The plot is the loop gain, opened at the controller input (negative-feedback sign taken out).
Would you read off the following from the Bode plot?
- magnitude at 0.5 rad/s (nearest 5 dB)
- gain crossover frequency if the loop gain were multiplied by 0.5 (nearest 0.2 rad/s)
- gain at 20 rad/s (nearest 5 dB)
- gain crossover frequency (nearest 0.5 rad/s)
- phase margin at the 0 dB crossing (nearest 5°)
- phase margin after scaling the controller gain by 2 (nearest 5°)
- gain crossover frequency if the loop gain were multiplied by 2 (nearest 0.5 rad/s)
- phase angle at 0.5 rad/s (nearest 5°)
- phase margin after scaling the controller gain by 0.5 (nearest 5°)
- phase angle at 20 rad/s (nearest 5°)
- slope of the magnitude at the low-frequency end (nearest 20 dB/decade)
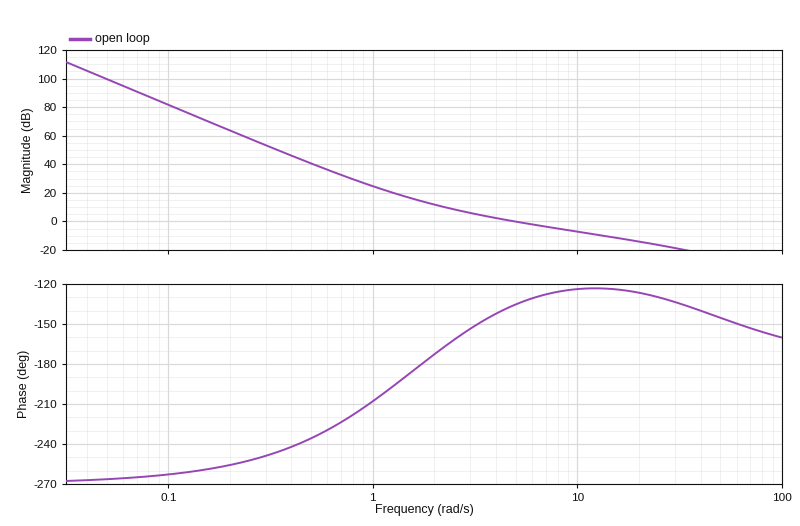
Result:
40 dB
3.0 rad/s
-15 dB
5.0 rad/s
45°
55°
9.0 rad/s
-235°
25°
-125°
-60 dB/decade
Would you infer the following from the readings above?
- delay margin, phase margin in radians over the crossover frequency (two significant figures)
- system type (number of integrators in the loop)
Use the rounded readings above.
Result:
0.16 s
3
